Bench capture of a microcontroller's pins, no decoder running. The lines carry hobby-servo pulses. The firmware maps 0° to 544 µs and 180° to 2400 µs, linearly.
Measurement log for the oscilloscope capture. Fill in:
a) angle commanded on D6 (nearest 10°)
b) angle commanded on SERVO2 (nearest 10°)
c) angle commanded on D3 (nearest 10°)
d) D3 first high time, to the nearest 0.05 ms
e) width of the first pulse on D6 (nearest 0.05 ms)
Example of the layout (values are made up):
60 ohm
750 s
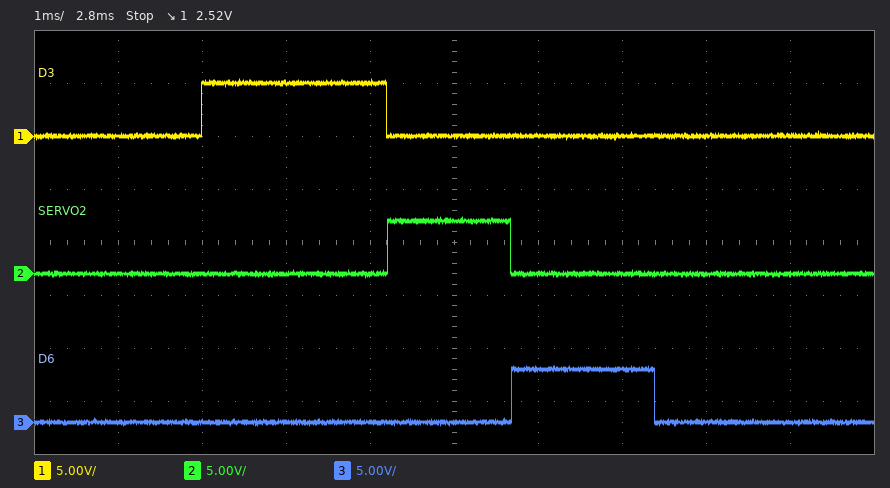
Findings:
110°
90°
160°
2.20 ms
1.70 ms
